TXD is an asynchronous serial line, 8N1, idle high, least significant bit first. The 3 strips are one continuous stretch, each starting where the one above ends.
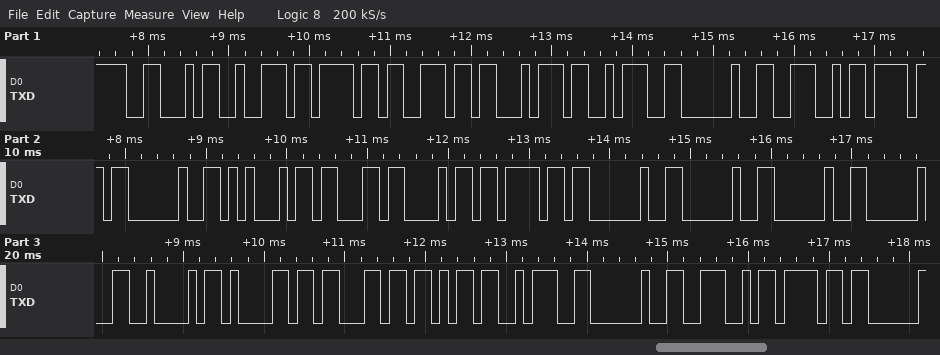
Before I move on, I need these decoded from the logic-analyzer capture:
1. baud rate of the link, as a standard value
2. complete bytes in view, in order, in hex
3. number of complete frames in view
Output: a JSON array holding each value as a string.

["9600 baud", "0x46 0x72 0x6F 0x6E 0x74 0x3A 0x20 0x4E 0x6F 0x20 0x45 0x63 0x68 0x6F 0x20 0x20 0x20 0x20 0x42 0x61 0x63 0x6B 0x3A 0x20 0x4E 0x6F", "26"]
